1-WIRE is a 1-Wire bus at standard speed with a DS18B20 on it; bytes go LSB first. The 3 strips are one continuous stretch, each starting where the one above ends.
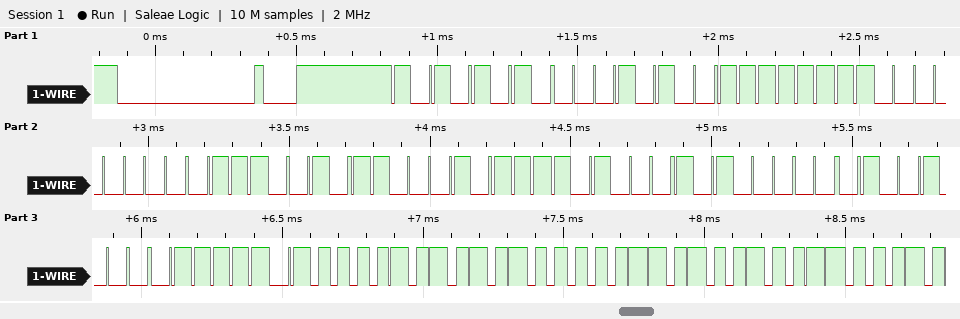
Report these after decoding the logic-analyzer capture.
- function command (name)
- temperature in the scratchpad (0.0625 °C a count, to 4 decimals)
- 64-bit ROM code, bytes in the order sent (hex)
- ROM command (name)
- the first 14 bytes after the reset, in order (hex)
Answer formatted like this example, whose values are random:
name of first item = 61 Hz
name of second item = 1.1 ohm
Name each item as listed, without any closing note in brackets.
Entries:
function command = Read Scratchpad
temperature in the scratchpad = 85.0000 °C
64-bit ROM code, bytes in the order sent = 28 FF 00 4E A3 17 05 12
ROM command = Match ROM
the first 14 bytes after the reset, in order = 55 28 FF 00 4E A3 17 05 12 BE 50 05 4B 46
